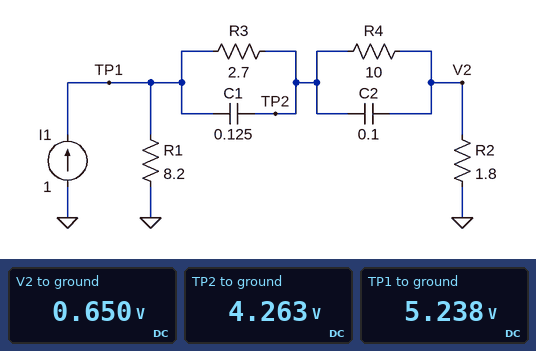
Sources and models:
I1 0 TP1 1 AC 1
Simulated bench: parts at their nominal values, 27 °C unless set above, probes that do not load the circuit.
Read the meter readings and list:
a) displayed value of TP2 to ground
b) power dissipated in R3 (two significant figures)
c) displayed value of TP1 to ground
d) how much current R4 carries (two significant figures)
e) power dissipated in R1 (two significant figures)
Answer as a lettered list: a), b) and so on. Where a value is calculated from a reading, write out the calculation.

a) 4.263 V
b) (5.238 V - 4.263 V)^2 / 2.7 Ω = 350 mW
c) 5.238 V
d) (4.263 V - 650 mV) / 10 Ω = 360 mA
e) (5.238 V)^2 / 8.2 Ω = 3.3 W
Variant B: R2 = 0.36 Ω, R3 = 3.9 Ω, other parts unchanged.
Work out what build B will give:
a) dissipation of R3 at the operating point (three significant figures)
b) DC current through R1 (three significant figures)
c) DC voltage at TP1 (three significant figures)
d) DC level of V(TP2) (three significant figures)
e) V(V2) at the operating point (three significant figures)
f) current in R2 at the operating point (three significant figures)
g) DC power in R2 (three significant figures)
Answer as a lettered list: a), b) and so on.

a) 520 mW
b) 635 mA
c) 5.21 V
d) 3.78 V
e) 131 mV
f) 365 mA
g) 48.0 mW
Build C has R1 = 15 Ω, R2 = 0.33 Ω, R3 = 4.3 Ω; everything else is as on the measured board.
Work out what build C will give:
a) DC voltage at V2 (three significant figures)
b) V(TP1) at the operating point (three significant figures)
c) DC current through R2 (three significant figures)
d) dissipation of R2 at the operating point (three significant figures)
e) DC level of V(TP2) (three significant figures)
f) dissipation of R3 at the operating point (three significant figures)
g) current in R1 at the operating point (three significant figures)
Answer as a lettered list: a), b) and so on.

a) 167 mV
b) 7.41 V
c) 506 mA
d) 84.6 mW
e) 5.23 V
f) 1.10 W
g) 494 mA
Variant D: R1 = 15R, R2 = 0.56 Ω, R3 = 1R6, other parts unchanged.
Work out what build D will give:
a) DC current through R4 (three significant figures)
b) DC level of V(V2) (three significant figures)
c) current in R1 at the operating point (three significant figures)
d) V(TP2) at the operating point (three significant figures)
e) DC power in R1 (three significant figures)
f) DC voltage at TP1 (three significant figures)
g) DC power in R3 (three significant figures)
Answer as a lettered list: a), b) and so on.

a) 552 mA
b) 309 mV
c) 448 mA
d) 5.83 V
e) 3.01 W
f) 6.72 V
g) 488 mW
